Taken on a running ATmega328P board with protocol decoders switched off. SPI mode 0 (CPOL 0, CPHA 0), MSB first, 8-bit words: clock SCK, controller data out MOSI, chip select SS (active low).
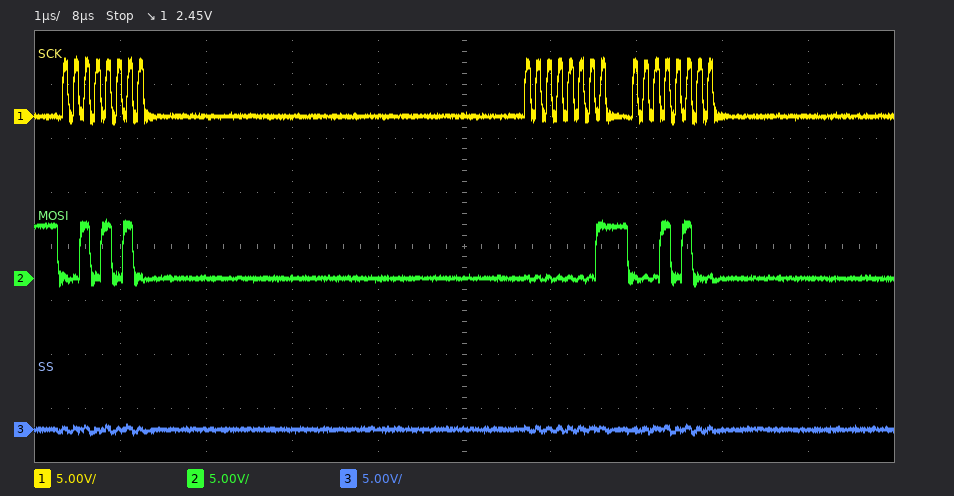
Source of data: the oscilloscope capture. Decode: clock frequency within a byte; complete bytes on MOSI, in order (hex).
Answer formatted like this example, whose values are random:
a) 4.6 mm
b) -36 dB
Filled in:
a) 8 MHz
b) 2A 01 14
